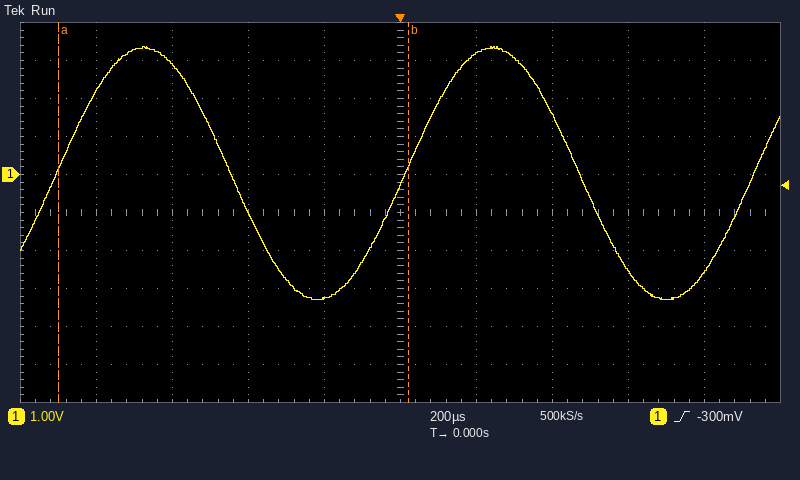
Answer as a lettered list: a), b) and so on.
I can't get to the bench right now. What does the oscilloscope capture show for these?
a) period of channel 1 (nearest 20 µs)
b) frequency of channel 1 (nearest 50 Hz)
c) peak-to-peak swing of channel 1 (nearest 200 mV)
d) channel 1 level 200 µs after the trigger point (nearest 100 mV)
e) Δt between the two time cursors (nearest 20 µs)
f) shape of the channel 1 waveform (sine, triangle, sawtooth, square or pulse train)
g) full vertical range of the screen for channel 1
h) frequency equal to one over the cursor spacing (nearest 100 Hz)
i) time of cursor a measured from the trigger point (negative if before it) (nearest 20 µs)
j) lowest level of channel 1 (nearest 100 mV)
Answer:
a) 920 µs
b) 1.10 kHz
c) 6.6 V
d) 3.2 V
e) 920 µs
f) sine
g) 10 V
h) 1.1 kHz
i) -900 µs
j) -3.3 V
